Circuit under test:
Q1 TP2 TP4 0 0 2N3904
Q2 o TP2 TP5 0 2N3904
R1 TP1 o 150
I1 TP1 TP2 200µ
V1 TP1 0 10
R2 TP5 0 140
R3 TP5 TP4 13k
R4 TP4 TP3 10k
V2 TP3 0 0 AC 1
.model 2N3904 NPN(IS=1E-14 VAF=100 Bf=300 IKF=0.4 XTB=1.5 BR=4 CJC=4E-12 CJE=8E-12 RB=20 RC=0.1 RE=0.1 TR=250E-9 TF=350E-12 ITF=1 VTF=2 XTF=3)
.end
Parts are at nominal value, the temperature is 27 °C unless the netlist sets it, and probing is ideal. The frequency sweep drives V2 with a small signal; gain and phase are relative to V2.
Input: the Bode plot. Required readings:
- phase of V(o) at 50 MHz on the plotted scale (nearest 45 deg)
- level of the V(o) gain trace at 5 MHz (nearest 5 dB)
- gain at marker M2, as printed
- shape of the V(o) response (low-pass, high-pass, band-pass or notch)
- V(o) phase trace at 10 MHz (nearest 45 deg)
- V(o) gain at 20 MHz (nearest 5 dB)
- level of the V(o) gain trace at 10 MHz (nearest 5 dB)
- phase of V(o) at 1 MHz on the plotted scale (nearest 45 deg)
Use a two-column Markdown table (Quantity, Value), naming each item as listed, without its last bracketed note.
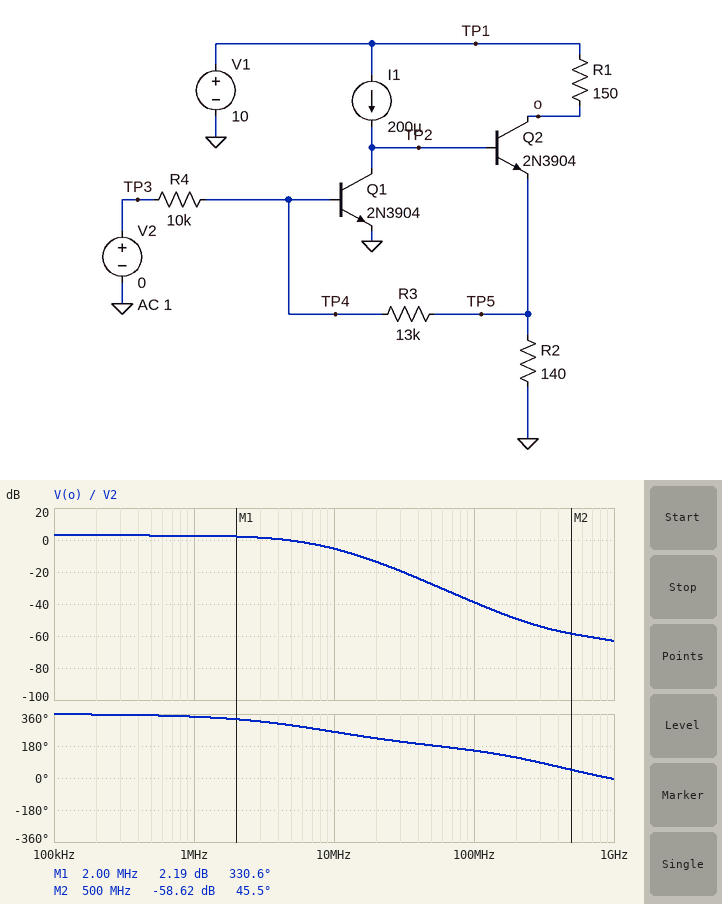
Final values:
| Quantity | Value |
|---|---|
| phase of V(o) at 50 MHz on the plotted scale | 180 deg |
| level of the V(o) gain trace at 5 MHz | 0 dB |
| gain at marker M2, as printed | -58.62 dB |
| shape of the V(o) response | low-pass |
| V(o) phase trace at 10 MHz | 270 deg |
| V(o) gain at 20 MHz | -15 dB |
| level of the V(o) gain trace at 10 MHz | -5 dB |
| phase of V(o) at 1 MHz on the plotted scale | 360 deg |
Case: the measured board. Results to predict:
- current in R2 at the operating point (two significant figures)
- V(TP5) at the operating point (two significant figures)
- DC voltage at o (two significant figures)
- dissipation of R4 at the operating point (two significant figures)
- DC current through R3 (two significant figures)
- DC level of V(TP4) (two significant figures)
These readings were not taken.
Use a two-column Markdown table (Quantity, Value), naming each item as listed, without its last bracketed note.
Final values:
| Quantity | Value |
|---|---|
| current in R2 at the operating point | 10 mA |
| V(TP5) at the operating point | 1.4 V |
| DC voltage at o | 8.5 V |
| dissipation of R4 at the operating point | 37 µW |
| DC current through R3 | 61 µA |
| DC level of V(TP4) | 610 mV |
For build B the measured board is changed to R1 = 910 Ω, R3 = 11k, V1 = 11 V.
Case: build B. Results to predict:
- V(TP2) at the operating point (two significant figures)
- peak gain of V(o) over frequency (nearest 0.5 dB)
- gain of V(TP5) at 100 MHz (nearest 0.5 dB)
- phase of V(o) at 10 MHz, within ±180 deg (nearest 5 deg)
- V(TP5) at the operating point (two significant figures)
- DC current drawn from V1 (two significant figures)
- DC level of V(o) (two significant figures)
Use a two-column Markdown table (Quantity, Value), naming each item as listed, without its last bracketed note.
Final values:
| Quantity | Value |
|---|---|
| V(TP2) at the operating point | 2.0 V |
| peak gain of V(o) over frequency | 17.0 dB |
| gain of V(TP5) at 100 MHz | -44.0 dB |
| phase of V(o) at 10 MHz, within ±180 deg | -140 deg |
| V(TP5) at the operating point | 1.3 V |
| DC current drawn from V1 | 9.4 mA |
| DC level of V(o) | 2.6 V |
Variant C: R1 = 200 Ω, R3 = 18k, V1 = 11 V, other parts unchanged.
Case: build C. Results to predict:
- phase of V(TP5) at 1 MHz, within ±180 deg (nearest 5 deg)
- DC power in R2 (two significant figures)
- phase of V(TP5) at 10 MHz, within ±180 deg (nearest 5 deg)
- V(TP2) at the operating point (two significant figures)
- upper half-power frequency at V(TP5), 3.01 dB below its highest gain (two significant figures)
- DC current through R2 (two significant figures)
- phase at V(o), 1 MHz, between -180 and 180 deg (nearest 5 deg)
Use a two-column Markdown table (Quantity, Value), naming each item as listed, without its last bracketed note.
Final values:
| Quantity | Value |
|---|---|
| phase of V(TP5) at 1 MHz, within ±180 deg | 160 deg |
| DC power in R2 | 21 mW |
| phase of V(TP5) at 10 MHz, within ±180 deg | 75 deg |
| V(TP2) at the operating point | 2.4 V |
| upper half-power frequency at V(TP5), 3.01 dB below its highest gain | 3.5 MHz |
| DC current through R2 | 12 mA |
| phase at V(o), 1 MHz, between -180 and 180 deg | -20 deg |
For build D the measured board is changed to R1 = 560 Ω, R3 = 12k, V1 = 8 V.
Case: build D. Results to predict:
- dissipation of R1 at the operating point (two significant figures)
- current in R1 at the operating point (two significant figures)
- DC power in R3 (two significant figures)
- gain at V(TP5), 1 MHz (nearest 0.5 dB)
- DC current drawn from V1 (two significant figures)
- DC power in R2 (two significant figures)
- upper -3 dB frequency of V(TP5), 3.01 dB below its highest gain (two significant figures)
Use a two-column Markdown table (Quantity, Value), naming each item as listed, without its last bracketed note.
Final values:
| Quantity | Value |
|---|---|
| dissipation of R1 at the operating point | 52 mW |
| current in R1 at the operating point | 9.6 mA |
| DC power in R3 | 45 µW |
| gain at V(TP5), 1 MHz | 1.5 dB |
| DC current drawn from V1 | 9.8 mA |
| DC power in R2 | 13 mW |
| upper -3 dB frequency of V(TP5), 3.01 dB below its highest gain | 5.0 MHz |
